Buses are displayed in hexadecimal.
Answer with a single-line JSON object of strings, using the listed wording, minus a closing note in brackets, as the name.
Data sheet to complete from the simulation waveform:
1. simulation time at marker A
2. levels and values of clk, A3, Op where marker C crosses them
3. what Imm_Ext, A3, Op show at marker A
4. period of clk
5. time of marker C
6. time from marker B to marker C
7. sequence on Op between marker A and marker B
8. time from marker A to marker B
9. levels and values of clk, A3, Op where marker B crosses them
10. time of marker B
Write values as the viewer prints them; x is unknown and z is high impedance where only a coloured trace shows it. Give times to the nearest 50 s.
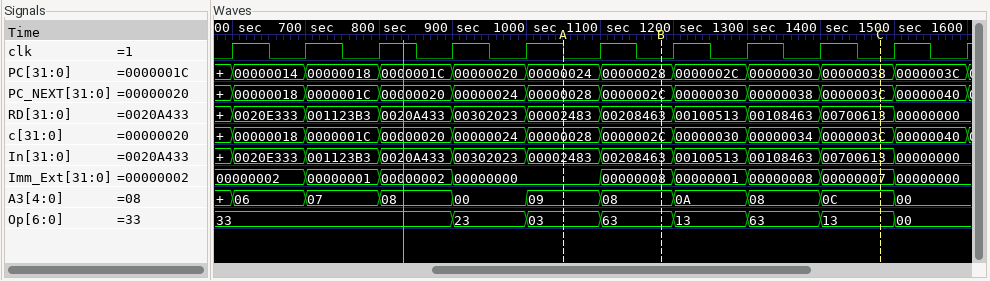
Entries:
{"simulation time at marker A": "1050 s", "levels and values of clk, A3, Op where marker C crosses them": "clk=0, A3=0C, Op=13", "what Imm_Ext, A3, Op show at marker A": "Imm_Ext=00000000, A3=09, Op=03", "period of clk": "100 s", "time of marker C": "1500 s", "time from marker B to marker C": "300 s", "sequence on Op between marker A and marker B": "03, 63", "time from marker A to marker B": "150 s", "levels and values of clk, A3, Op where marker B crosses them": "clk=0, A3=08, Op=63", "time of marker B": "1200 s"}
